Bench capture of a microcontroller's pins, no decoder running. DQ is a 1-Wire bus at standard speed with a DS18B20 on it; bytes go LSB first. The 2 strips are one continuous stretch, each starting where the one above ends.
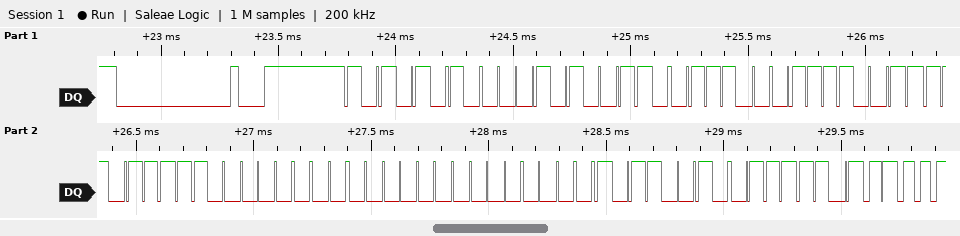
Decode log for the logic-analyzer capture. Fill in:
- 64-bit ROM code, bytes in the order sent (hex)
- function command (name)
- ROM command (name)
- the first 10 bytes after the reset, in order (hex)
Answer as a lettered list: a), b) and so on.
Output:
a) 28 73 3C EF 03 00 00 4D
b) Read Scratchpad
c) Match ROM
d) 55 28 73 3C EF 03 00 00 4D BE
